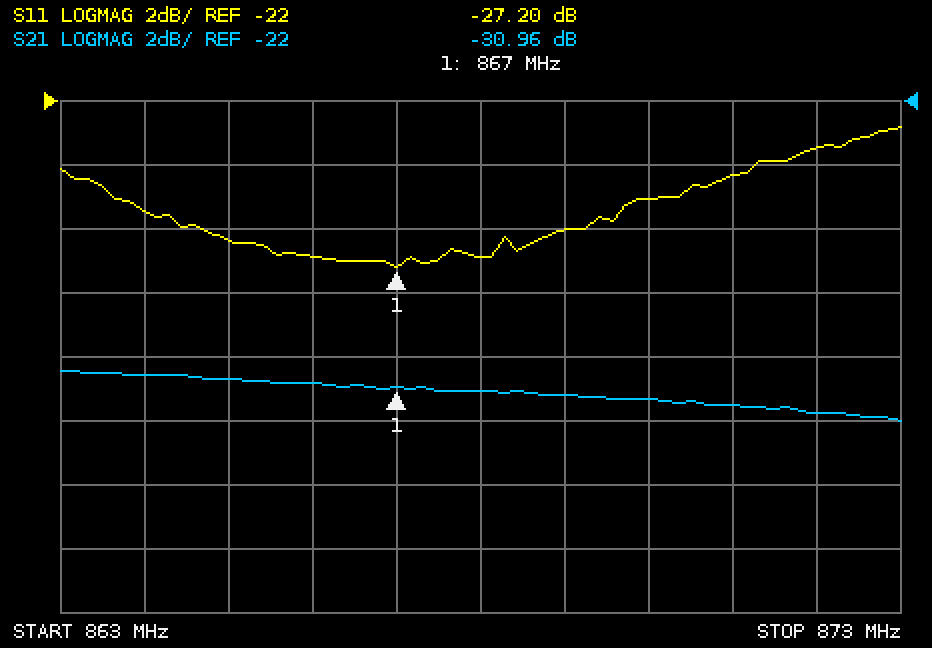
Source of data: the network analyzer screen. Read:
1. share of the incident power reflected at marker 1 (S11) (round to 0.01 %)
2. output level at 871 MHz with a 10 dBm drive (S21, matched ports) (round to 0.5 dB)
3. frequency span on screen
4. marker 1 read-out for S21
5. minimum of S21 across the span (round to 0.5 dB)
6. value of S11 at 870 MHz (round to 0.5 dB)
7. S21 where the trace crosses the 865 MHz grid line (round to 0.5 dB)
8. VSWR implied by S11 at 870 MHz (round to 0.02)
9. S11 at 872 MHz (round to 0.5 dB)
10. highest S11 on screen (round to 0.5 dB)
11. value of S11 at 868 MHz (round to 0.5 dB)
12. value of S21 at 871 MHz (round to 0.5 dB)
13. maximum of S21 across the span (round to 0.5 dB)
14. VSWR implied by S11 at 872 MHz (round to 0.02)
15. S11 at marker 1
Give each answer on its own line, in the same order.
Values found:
0.19 %
-21.5 dBm
10 MHz
-30.96 dB
-32.0 dB
-25.0 dB
-30.5 dB
1.12
-23.5 dB
-23.0 dB
-27.0 dB
-31.5 dB
-30.5 dB
1.14
-27.20 dB
